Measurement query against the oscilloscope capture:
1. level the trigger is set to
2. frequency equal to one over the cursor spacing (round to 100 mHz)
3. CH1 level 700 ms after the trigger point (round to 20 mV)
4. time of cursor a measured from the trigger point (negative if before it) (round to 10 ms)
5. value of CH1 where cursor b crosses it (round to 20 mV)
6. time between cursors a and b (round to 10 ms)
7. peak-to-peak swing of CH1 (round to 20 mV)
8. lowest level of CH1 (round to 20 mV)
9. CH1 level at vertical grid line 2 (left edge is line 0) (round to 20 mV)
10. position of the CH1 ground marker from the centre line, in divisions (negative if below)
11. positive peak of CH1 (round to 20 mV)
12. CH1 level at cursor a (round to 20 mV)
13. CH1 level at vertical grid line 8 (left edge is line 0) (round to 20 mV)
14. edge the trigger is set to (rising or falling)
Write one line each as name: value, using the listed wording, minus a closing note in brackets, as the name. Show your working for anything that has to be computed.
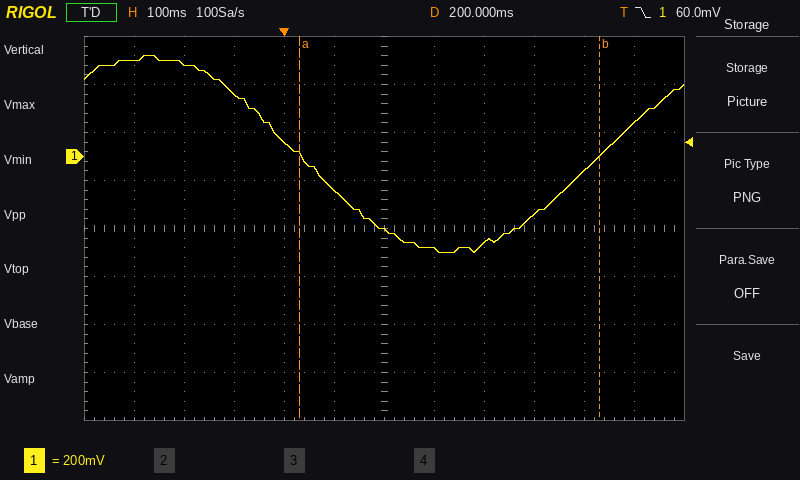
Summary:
level the trigger is set to: 60.0 mV
frequency equal to one over the cursor spacing: 1 / 600 ms ≈ 1.7 Hz
CH1 level 700 ms after the trigger point: 140 mV
time of cursor a measured from the trigger point (negative if before it): +30 ms
value of CH1 where cursor b crosses it: 0 mV
time between cursors a and b: 600 ms
peak-to-peak swing of CH1: 420 mV − (-400 mV) = 820 mV
lowest level of CH1: -400 mV
CH1 level at vertical grid line 2 (left edge is line 0): 380 mV
position of the CH1 ground marker from the centre line, in divisions: +1.5 div
positive peak of CH1: 420 mV
CH1 level at cursor a: 0 mV
CH1 level at vertical grid line 8 (left edge is line 0): -360 mV
edge the trigger is set to: falling
